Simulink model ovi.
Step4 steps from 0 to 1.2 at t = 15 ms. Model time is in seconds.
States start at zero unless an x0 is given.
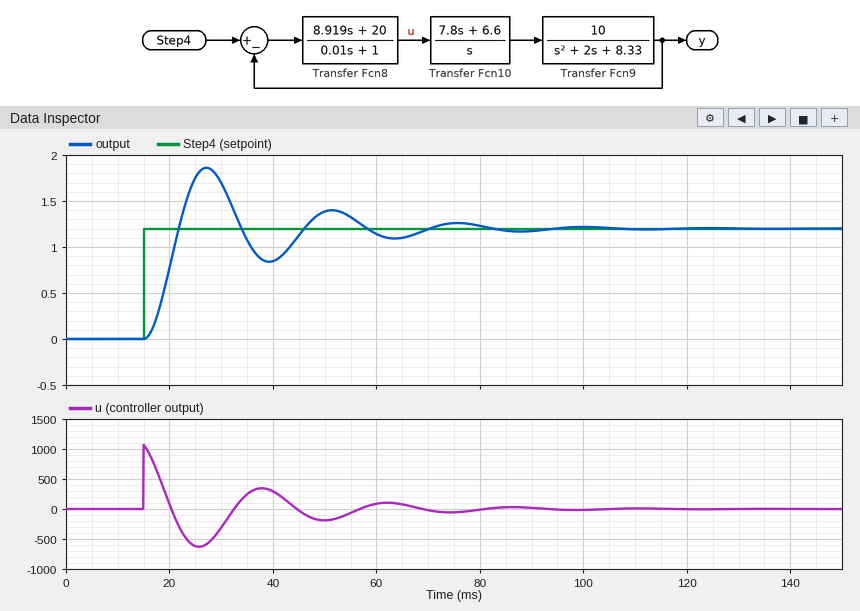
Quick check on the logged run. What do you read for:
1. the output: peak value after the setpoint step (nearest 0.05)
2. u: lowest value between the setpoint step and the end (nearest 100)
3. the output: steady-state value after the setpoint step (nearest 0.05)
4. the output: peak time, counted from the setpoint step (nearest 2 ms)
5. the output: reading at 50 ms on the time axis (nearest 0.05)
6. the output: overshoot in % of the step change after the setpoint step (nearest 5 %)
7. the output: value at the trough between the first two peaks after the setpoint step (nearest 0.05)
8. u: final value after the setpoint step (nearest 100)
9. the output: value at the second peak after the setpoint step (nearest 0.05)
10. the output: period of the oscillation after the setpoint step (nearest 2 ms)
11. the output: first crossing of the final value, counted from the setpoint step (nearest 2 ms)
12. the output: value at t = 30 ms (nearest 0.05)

1.85
-600
1.20
12 ms
1.40
55 %
0.85
0
1.40
24 ms
6 ms
1.70
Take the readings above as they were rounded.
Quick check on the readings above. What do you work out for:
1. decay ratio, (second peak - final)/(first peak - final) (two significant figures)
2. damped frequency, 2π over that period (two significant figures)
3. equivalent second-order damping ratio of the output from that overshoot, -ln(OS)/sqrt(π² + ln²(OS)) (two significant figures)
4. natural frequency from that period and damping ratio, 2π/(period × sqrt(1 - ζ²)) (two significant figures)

0.31
0.26 rad/ms
0.19
0.27 rad/ms
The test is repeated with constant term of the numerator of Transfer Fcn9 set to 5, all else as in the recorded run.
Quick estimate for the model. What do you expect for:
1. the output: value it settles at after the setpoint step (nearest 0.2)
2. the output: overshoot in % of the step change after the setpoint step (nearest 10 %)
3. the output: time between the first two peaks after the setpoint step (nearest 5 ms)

1.2
40 %
35 ms
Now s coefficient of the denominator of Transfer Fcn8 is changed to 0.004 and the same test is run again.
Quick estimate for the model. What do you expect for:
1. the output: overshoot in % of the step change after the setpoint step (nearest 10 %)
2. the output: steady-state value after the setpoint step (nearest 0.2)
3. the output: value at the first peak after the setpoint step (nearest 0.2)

40 %
1.2
1.6
